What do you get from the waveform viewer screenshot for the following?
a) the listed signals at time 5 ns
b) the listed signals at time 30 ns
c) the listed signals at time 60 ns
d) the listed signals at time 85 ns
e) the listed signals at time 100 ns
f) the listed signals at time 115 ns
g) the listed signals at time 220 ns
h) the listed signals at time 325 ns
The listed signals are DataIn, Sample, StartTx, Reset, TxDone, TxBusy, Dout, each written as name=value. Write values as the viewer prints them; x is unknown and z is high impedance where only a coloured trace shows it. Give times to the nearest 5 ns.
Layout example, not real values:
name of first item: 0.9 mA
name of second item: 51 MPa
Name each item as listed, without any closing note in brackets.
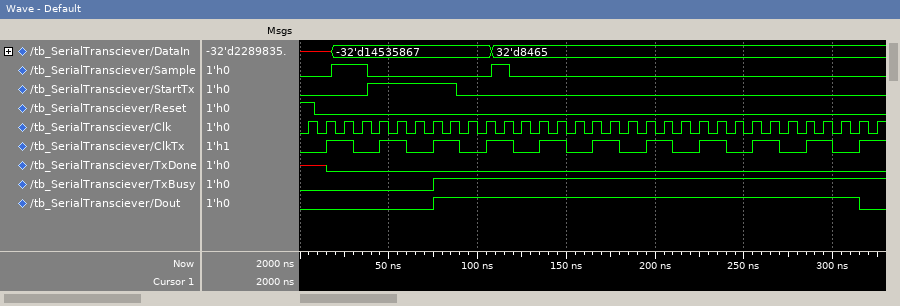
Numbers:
the listed signals at time 5 ns: DataIn=x, Sample=0, StartTx=0, Reset=1, TxDone=x, TxBusy=0, Dout=0
the listed signals at time 30 ns: DataIn=-32'd14535867, Sample=1, StartTx=0, Reset=0, TxDone=0, TxBusy=0, Dout=0
the listed signals at time 60 ns: DataIn=-32'd14535867, Sample=0, StartTx=1, Reset=0, TxDone=0, TxBusy=0, Dout=0
the listed signals at time 85 ns: DataIn=-32'd14535867, Sample=0, StartTx=1, Reset=0, TxDone=0, TxBusy=1, Dout=1
the listed signals at time 100 ns: DataIn=-32'd14535867, Sample=0, StartTx=0, Reset=0, TxDone=0, TxBusy=1, Dout=1
the listed signals at time 115 ns: DataIn=32'd8465, Sample=1, StartTx=0, Reset=0, TxDone=0, TxBusy=1, Dout=1
the listed signals at time 220 ns: DataIn=32'd8465, Sample=0, StartTx=0, Reset=0, TxDone=0, TxBusy=1, Dout=1
the listed signals at time 325 ns: DataIn=32'd8465, Sample=0, StartTx=0, Reset=0, TxDone=0, TxBusy=1, Dout=0
